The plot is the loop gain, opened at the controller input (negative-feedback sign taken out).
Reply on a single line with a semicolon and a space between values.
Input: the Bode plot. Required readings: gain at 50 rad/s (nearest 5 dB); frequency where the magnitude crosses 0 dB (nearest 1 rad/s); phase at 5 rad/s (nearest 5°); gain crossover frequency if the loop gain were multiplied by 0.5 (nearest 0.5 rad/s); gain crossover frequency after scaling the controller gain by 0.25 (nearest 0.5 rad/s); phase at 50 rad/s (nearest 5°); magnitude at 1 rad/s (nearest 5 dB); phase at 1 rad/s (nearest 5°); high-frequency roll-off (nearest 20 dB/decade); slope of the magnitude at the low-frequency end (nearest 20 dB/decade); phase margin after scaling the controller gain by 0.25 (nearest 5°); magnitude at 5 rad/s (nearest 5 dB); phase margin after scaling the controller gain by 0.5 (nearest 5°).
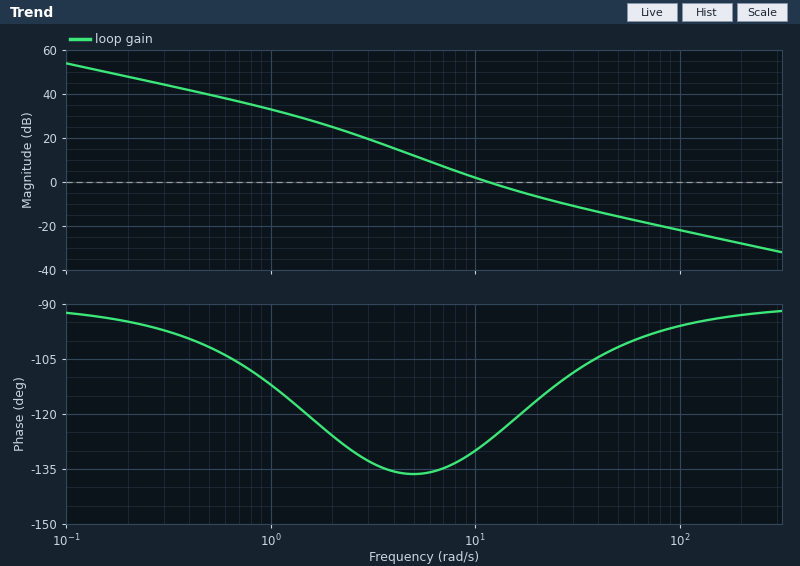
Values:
-15 dB; 12 rad/s; -135°; 7.5 rad/s; 5.0 rad/s; -100°; 35 dB; -110°; -20 dB/decade; -20 dB/decade; 45°; 10 dB; 45°
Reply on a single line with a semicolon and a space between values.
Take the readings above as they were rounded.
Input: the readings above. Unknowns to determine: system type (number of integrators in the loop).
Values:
1
